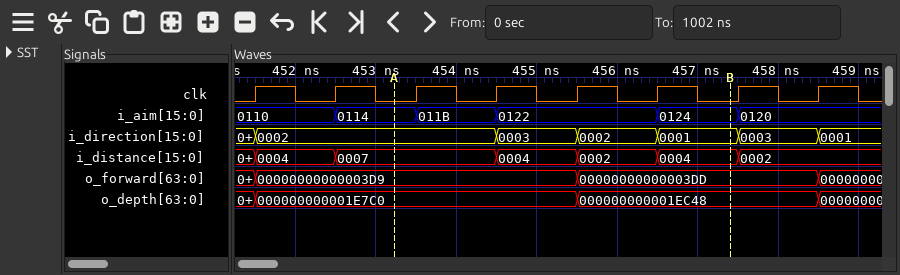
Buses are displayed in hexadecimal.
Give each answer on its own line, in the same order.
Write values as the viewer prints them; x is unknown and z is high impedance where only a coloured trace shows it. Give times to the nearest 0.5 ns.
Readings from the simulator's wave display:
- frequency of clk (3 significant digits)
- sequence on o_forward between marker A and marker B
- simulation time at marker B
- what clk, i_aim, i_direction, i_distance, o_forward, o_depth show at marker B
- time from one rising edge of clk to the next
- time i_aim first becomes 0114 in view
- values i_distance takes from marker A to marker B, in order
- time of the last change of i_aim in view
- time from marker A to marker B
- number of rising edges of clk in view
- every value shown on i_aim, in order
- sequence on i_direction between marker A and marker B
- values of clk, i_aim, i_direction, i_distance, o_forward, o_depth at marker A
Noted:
1.00 GHz
00000000000003D9, 00000000000003DD
457.5 ns
clk=0, i_aim=0124, i_direction=0001, i_distance=0004, o_forward=00000000000003DD, o_depth=000000000001EC48
1 ns
452.5 ns
0007, 0004, 0002, 0004
457.5 ns
4 ns
8
0110, 0114, 011B, 0122, 0124, 0120
0002, 0003, 0002, 0001
clk=0, i_aim=0114, i_direction=0002, i_distance=0007, o_forward=00000000000003D9, o_depth=000000000001E7C0
